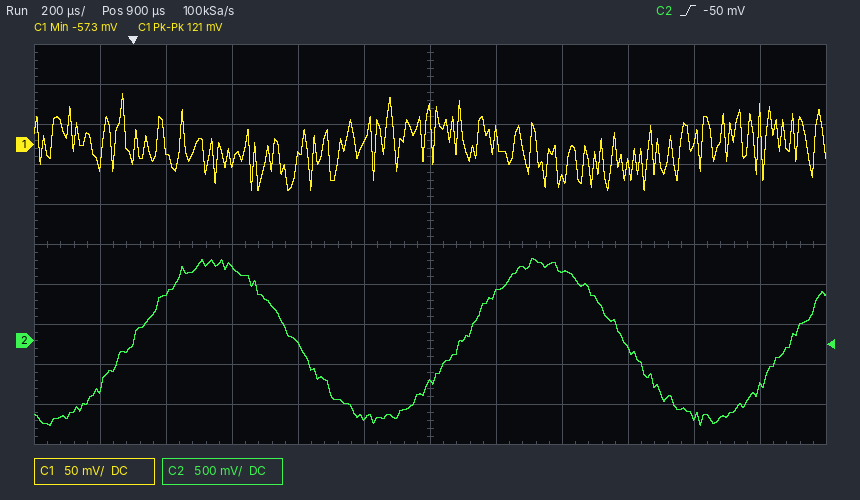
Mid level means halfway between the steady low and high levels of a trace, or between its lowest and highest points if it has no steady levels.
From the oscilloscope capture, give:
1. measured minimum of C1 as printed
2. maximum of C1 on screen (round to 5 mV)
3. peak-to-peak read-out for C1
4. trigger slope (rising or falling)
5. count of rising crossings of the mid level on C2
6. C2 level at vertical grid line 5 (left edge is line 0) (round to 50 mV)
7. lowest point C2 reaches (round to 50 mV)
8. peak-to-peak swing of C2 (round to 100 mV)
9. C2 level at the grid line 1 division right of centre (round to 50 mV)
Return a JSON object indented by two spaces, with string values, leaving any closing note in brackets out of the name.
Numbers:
{
  "measured minimum of C1 as printed": "-57.3 mV",
  "maximum of C1 on screen": "65 mV",
  "peak-to-peak read-out for C1": "121 mV",
  "trigger slope": "rising",
  "count of rising crossings of the mid level on C2": "3",
  "C2 level at vertical grid line 5 (left edge is line 0)": "-950 mV",
  "lowest point C2 reaches": "-1.05 V",
  "peak-to-peak swing of C2": "2.10 V",
  "C2 level at the grid line 1 division right of centre": "600 mV"
}
